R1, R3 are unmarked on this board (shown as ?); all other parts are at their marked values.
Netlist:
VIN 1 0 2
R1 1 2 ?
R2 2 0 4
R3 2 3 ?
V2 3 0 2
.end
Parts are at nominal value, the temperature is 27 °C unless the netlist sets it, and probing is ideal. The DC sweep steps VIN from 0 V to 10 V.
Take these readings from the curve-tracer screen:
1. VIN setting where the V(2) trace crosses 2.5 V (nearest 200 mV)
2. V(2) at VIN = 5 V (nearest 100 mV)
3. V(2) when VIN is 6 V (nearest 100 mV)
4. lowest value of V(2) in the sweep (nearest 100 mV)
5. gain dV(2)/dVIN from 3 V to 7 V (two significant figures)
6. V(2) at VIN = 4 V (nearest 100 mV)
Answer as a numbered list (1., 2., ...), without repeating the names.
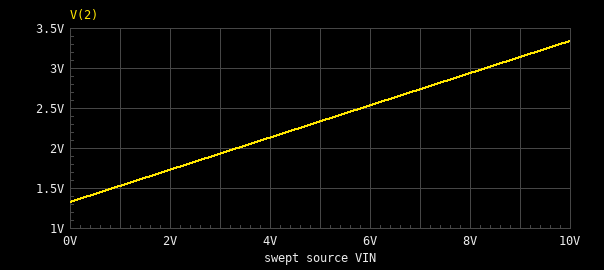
1. 5.8 V
2. 2.3 V
3. 2.5 V
4. 1.3 V
5. 0.20 V/V
6. 2.1 V
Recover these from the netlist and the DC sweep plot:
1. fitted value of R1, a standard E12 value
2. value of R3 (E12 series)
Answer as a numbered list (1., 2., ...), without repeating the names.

1. 2.7 Ω
2. 0.82 Ω
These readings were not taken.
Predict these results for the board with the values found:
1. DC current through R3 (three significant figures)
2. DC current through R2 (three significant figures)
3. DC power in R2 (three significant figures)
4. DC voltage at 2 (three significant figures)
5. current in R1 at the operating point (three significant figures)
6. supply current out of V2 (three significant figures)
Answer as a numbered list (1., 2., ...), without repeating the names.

1. 331 mA
2. 432 mA
3. 747 mW
4. 1.73 V
5. 101 mA
6. 331 mA
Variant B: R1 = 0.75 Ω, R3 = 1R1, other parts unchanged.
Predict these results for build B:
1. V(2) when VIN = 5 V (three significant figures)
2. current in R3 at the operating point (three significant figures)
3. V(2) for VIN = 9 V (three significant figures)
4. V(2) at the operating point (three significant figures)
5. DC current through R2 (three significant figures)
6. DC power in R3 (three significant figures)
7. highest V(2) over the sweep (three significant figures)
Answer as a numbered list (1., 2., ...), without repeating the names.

1. 3.40 V
2. 182 mA
3. 5.54 V
4. 1.80 V
5. 450 mA
6. 36.6 mW
7. 6.08 V
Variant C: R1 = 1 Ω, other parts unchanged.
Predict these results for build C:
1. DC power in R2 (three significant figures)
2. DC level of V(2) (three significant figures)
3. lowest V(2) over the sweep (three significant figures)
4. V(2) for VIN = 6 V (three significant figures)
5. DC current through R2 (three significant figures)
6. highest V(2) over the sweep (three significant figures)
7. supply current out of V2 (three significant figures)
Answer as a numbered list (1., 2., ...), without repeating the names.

1. 808 mW
2. 1.80 V
3. 988 mV
4. 3.42 V
5. 449 mA
6. 5.04 V
7. 247 mA
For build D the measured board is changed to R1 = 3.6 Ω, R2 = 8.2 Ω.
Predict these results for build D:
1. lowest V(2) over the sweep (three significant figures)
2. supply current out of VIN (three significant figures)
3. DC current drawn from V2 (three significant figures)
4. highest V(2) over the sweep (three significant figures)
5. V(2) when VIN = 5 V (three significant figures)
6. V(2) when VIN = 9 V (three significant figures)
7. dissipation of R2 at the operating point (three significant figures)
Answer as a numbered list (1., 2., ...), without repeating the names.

1. 1.51 V
2. 41.8 mA
3. 184 mA
4. 3.22 V
5. 2.36 V
6. 3.05 V
7. 417 mW
